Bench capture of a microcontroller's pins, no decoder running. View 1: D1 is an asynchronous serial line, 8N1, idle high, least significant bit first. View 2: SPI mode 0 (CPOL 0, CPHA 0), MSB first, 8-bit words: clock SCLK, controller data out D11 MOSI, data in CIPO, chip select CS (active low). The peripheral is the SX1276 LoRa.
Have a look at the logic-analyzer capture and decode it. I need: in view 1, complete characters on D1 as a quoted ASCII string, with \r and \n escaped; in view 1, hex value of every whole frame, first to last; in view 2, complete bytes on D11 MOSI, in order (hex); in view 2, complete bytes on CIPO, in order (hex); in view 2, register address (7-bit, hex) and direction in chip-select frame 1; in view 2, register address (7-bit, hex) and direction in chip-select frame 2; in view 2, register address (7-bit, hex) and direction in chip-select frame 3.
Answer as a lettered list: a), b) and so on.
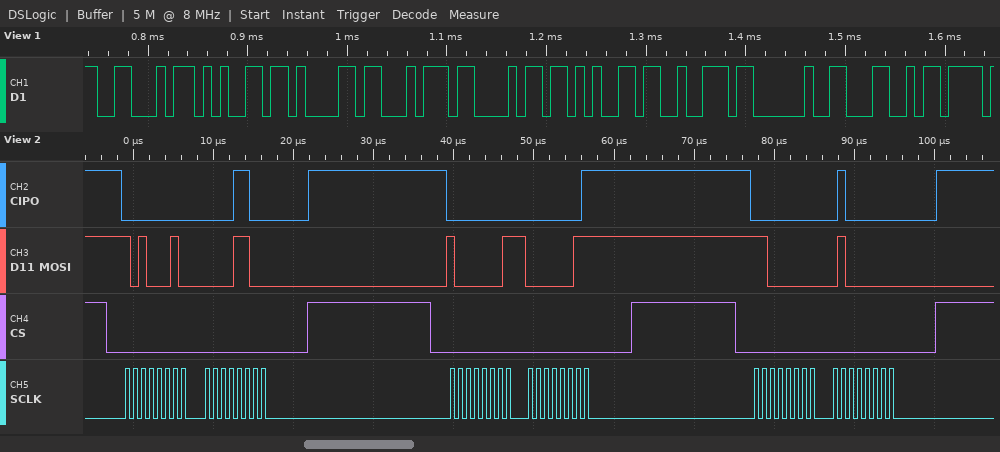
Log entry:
a) "Feather L"
b) 46 65 61 74 68 65 72 20 4C
c) A2 0C 81 03 C0 40
d) 00 0C 00 01 00 40
e) 0x22 write
f) 0x01 write
g) 0x40 write
